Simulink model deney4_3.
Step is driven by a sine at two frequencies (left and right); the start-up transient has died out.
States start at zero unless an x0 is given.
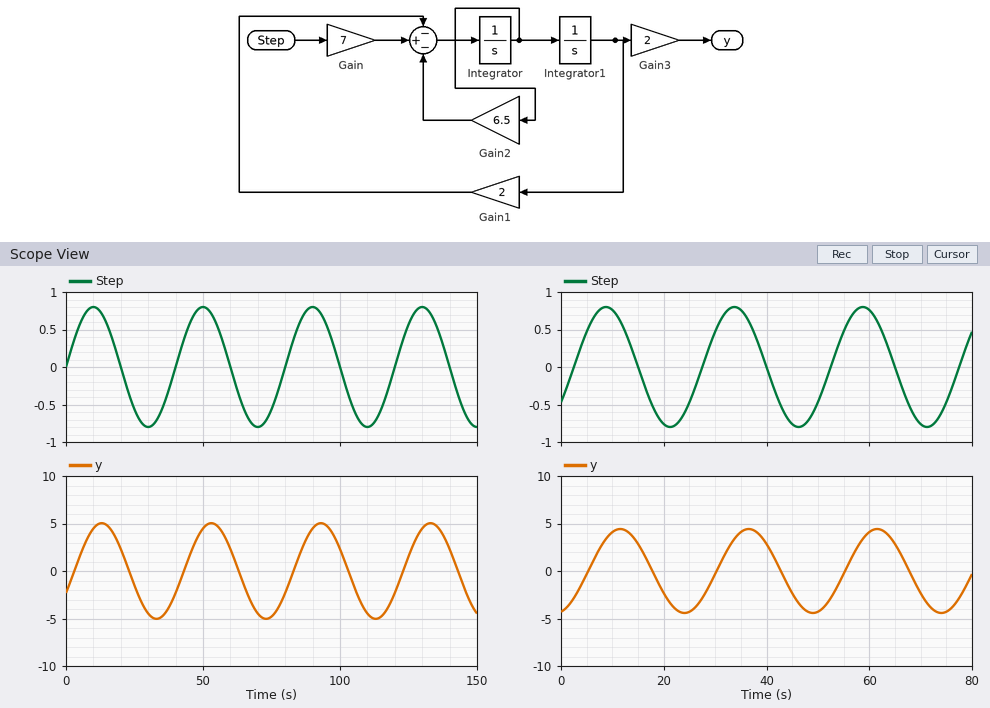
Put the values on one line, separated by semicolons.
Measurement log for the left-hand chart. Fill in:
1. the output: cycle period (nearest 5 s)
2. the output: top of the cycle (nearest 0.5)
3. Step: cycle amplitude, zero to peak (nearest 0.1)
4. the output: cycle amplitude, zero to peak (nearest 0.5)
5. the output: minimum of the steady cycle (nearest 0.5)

40 s; 5.0; 0.8; 5.0; -5.0
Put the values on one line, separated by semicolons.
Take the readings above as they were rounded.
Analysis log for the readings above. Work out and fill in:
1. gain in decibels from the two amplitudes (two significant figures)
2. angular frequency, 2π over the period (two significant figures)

16 dB; 0.16 rad/s
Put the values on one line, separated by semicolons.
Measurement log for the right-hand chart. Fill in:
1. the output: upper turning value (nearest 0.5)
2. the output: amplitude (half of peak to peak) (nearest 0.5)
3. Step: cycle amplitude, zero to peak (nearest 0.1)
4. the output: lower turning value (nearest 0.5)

4.5; 4.5; 0.8; -4.5
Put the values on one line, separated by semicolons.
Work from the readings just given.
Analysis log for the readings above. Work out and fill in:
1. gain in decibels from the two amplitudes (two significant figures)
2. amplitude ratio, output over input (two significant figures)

15 dB; 5.6
